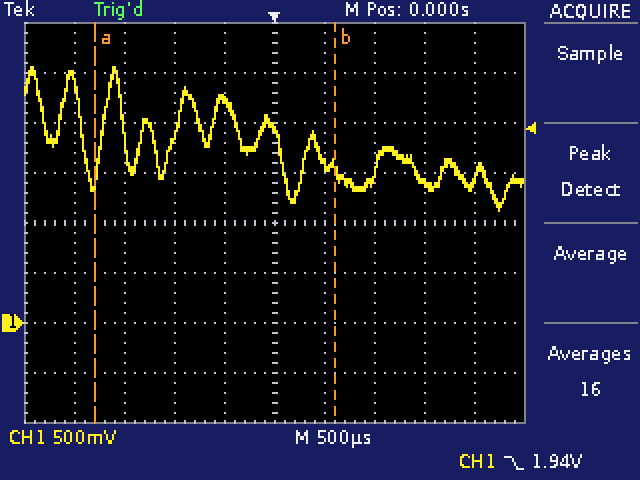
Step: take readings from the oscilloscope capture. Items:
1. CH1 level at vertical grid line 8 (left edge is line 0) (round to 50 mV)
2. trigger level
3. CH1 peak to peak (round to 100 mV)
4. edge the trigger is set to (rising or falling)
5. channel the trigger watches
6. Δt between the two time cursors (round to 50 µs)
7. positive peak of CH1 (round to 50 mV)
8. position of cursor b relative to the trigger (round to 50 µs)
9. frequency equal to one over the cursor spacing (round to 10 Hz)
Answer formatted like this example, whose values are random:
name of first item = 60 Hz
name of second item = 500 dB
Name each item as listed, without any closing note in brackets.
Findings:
CH1 level at vertical grid line 8 (left edge is line 0) = 1.40 V
trigger level = 1.94 V
CH1 peak to peak = 1.40 V
edge the trigger is set to = falling
channel the trigger watches = CH1
Δt between the two time cursors = 2.40 ms
positive peak of CH1 = 2.55 V
position of cursor b relative to the trigger = +600 µs
frequency equal to one over the cursor spacing = 420 Hz
